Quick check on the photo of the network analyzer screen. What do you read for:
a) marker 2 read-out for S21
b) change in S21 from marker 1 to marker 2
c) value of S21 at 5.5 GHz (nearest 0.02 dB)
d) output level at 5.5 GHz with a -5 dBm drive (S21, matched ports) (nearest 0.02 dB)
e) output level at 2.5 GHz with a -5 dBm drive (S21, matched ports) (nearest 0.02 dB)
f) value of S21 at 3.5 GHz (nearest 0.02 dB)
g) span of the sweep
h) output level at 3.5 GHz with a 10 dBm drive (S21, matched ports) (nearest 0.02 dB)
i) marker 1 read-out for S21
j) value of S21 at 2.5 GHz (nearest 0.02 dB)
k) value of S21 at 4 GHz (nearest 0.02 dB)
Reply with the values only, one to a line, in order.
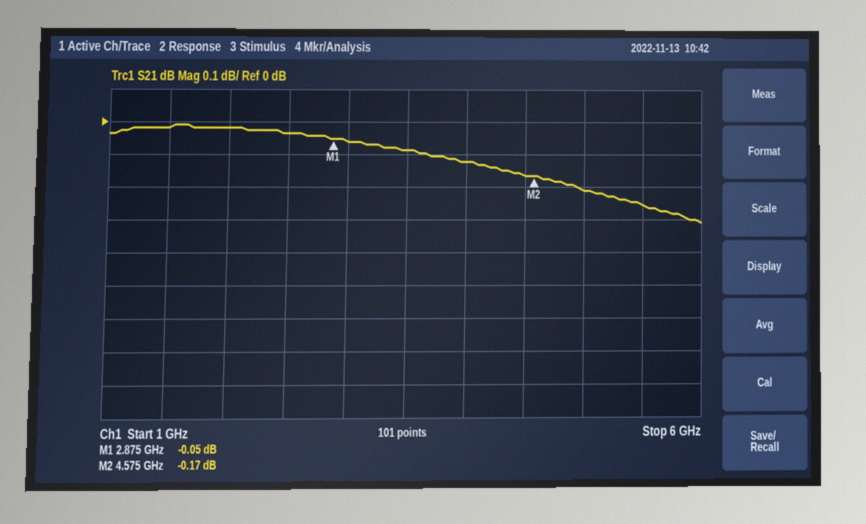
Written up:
-0.17 dB
-0.12 dB
-0.26 dB
-5.26 dBm
-5.04 dBm
-0.08 dB
5 GHz
9.92 dBm
-0.05 dB
-0.04 dB
-0.12 dB
